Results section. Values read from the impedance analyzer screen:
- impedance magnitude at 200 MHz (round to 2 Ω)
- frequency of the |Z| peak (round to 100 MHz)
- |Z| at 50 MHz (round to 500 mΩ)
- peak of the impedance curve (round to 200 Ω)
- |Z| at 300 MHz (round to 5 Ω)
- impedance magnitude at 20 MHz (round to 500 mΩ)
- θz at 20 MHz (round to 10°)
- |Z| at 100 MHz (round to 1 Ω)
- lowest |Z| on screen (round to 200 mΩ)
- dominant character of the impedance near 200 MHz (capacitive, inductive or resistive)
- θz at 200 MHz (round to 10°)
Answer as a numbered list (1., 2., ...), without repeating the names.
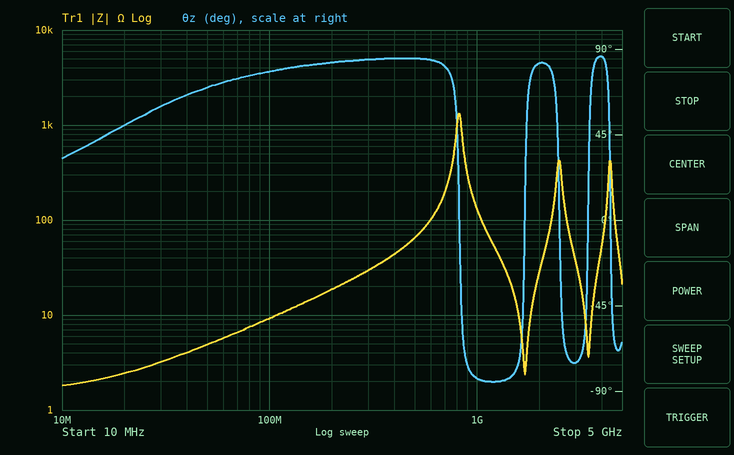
1. 18 Ω
2. 800 MHz
3. 5.0 Ω
4. 1.4 kΩ
5. 30 Ω
6. 2.5 Ω
7. 50°
8. 9 Ω
9. 1.8 Ω
10. inductive
11. 80°
